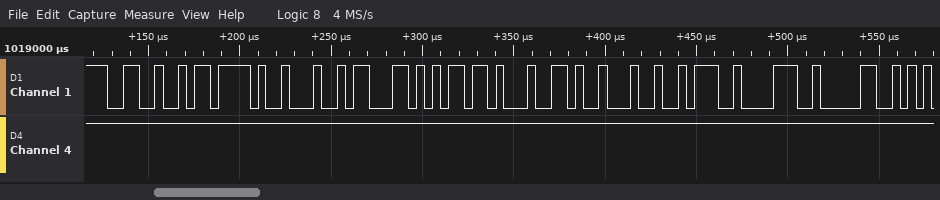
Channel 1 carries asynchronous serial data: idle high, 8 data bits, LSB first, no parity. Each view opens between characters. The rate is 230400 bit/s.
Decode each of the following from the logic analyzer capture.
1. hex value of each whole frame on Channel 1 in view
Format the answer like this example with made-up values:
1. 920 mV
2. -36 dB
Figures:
1. 26, 7B, 22, 63, 6D, 64, 22, 3A, 38, 30
